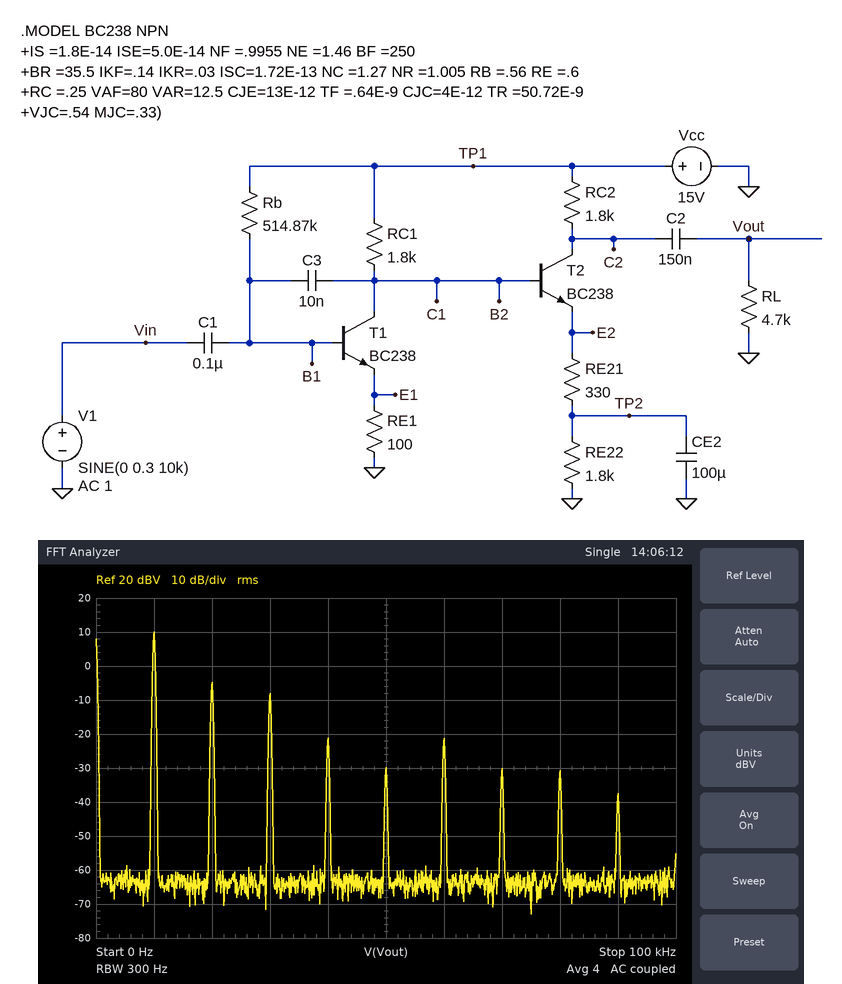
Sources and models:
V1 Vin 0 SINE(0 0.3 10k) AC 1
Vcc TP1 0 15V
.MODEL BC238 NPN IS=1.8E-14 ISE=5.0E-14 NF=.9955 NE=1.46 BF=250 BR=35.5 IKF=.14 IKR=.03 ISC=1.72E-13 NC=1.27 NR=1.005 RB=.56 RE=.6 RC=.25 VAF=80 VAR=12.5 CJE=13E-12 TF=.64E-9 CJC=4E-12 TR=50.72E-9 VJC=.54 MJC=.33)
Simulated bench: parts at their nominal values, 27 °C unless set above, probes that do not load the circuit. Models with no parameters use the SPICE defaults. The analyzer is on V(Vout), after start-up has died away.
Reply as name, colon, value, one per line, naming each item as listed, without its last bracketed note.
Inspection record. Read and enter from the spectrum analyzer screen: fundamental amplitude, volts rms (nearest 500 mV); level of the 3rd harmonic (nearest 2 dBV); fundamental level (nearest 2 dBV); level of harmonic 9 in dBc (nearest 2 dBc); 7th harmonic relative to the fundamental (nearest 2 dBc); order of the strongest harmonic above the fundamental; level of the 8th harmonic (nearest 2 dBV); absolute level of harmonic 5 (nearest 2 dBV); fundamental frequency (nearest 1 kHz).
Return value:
fundamental amplitude, volts rms: 3.0 V
level of the 3rd harmonic: -8 dBV
fundamental level: 10 dBV
level of harmonic 9 in dBc: -48 dBc
7th harmonic relative to the fundamental: -40 dBc
order of the strongest harmonic above the fundamental: 2
level of the 8th harmonic: -30 dBV
absolute level of harmonic 5: -30 dBV
fundamental frequency: 10 kHz
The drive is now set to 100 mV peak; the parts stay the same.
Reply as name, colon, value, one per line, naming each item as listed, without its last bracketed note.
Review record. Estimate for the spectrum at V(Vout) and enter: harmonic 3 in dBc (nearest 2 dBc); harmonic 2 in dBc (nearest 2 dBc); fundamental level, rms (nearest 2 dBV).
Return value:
harmonic 3 in dBc: -50 dBc
harmonic 2 in dBc: -40 dBc
fundamental level, rms: 4 dBV
